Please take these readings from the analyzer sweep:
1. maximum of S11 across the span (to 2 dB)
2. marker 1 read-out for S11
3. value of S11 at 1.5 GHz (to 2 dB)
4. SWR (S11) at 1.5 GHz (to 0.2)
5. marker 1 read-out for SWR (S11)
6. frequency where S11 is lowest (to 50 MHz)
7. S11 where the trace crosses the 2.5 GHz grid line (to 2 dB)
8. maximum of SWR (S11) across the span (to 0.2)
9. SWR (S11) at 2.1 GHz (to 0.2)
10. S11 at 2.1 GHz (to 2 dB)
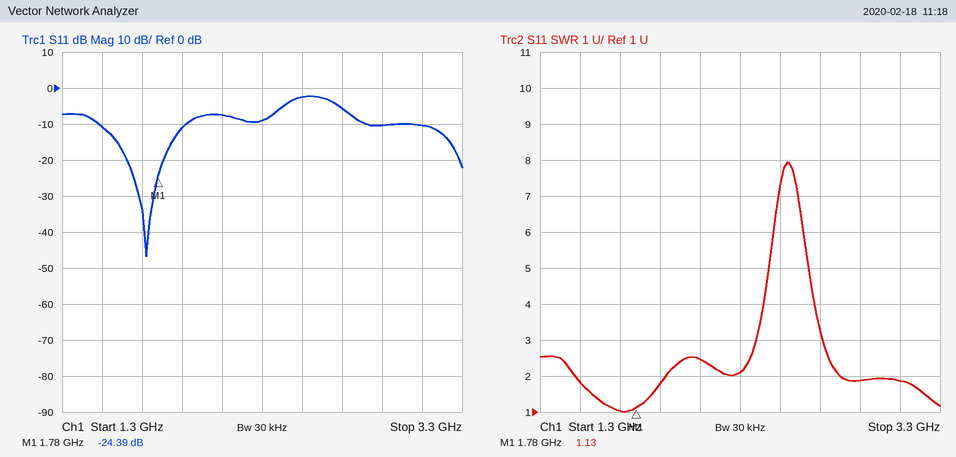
-2 dB
-24.39 dB
-10 dB
1.8
1.13
1.70 GHz
-2 dB
8.0
2.4
-8 dB
